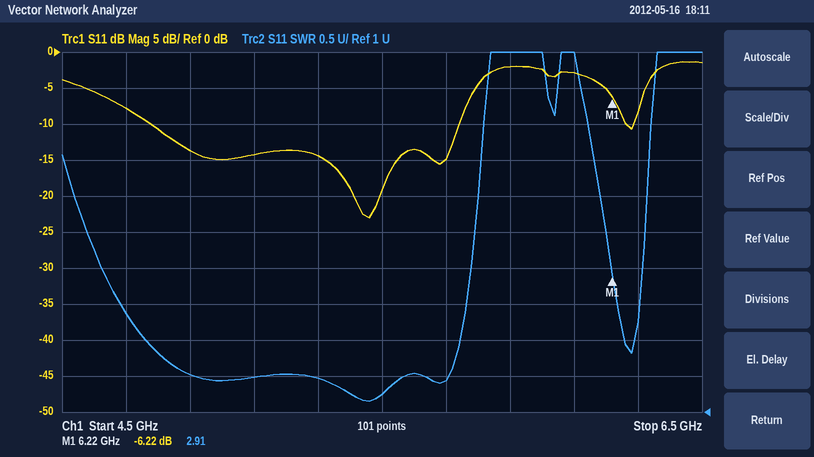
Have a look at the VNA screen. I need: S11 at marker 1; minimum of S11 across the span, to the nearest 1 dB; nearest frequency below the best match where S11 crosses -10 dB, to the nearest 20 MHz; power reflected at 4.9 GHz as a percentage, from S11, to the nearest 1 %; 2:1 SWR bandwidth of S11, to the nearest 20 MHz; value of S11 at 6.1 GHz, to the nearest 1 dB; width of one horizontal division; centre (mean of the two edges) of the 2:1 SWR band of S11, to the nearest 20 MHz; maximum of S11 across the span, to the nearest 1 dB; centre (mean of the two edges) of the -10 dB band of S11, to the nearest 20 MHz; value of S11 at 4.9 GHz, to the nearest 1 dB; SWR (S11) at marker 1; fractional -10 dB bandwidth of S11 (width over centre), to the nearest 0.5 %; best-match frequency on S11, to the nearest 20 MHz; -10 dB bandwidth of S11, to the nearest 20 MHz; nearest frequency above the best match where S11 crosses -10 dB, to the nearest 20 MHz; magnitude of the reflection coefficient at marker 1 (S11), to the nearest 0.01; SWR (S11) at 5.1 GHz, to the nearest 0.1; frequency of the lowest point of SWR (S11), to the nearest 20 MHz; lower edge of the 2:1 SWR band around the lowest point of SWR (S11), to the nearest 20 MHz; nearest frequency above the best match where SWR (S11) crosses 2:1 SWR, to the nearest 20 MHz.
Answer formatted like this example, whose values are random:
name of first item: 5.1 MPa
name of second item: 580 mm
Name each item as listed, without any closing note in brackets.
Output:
S11 at marker 1: -6.22 dB
minimum of S11 across the span, to the nearest 1 dB: -23 dB
nearest frequency below the best match where S11 crosses -10 dB, to the nearest 20 MHz: 4.78 GHz
power reflected at 4.9 GHz as a percentage, from S11, to the nearest 1 %: 4 %
2:1 SWR bandwidth of S11, to the nearest 20 MHz: 980 MHz
value of S11 at 6.1 GHz, to the nearest 1 dB: -3 dB
width of one horizontal division: 200 MHz
centre (mean of the two edges) of the 2:1 SWR band of S11, to the nearest 20 MHz: 5.26 GHz
maximum of S11 across the span, to the nearest 1 dB: -1 dB
centre (mean of the two edges) of the -10 dB band of S11, to the nearest 20 MHz: 5.26 GHz
value of S11 at 4.9 GHz, to the nearest 1 dB: -14 dB
SWR (S11) at marker 1: 2.91
fractional -10 dB bandwidth of S11 (width over centre), to the nearest 0.5 %: 18.5 %
best-match frequency on S11, to the nearest 20 MHz: 5.46 GHz
-10 dB bandwidth of S11, to the nearest 20 MHz: 960 MHz
nearest frequency above the best match where S11 crosses -10 dB, to the nearest 20 MHz: 5.74 GHz
magnitude of the reflection coefficient at marker 1 (S11), to the nearest 0.01: 0.49
SWR (S11) at 5.1 GHz, to the nearest 0.1: 1.5
frequency of the lowest point of SWR (S11), to the nearest 20 MHz: 5.46 GHz
lower edge of the 2:1 SWR band around the lowest point of SWR (S11), to the nearest 20 MHz: 4.76 GHz
nearest frequency above the best match where SWR (S11) crosses 2:1 SWR, to the nearest 20 MHz: 5.74 GHz
